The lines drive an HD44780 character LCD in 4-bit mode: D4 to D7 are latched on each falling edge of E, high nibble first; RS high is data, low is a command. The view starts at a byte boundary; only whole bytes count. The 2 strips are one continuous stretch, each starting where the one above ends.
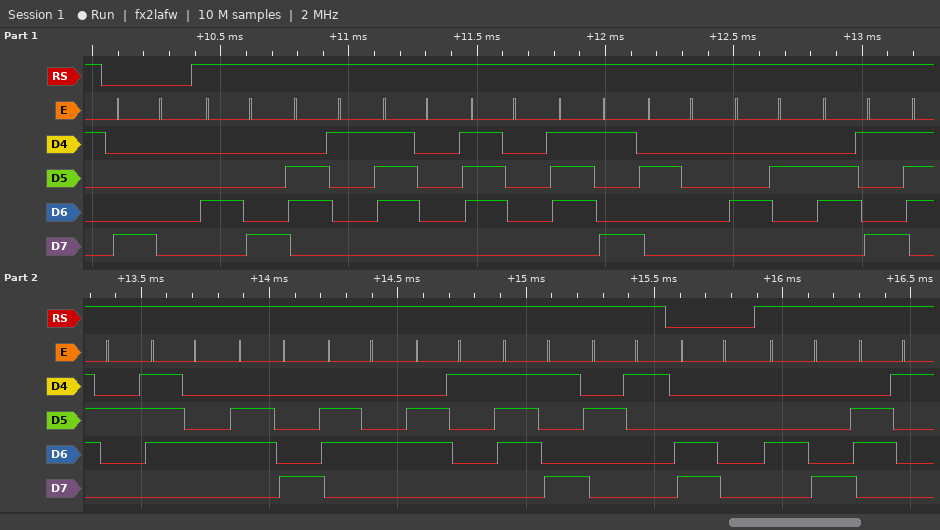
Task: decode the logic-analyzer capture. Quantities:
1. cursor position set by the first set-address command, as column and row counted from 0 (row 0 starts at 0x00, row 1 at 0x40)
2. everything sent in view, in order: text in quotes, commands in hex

column 0, row 0
0x80 "Happy Birthday!" 0xC0 "Ha"
